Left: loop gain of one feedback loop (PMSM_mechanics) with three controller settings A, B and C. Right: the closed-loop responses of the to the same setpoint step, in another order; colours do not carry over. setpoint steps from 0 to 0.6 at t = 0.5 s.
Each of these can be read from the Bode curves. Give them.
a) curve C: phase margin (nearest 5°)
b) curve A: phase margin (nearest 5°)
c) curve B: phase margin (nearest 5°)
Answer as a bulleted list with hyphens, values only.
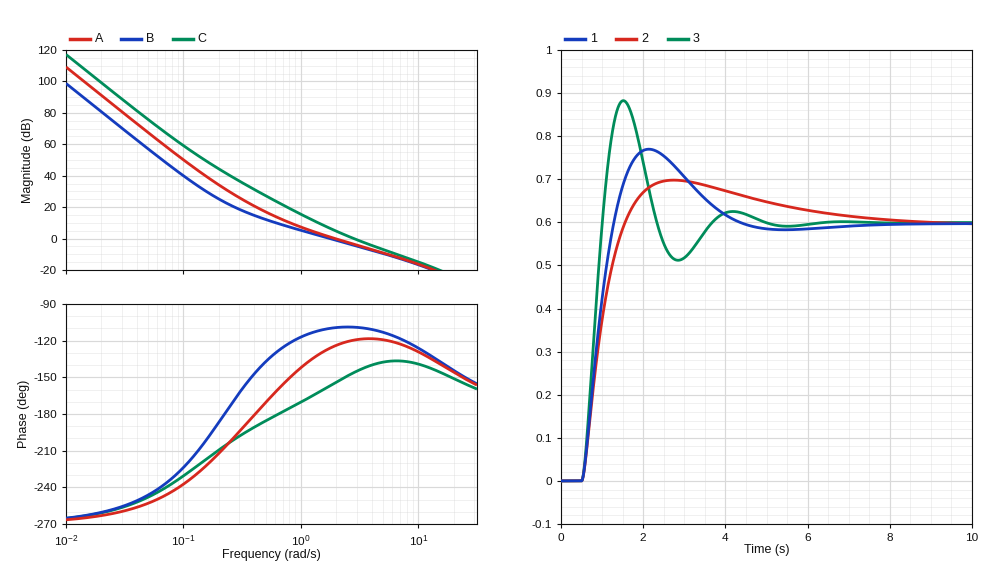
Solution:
- 35°
- 55°
- 70°
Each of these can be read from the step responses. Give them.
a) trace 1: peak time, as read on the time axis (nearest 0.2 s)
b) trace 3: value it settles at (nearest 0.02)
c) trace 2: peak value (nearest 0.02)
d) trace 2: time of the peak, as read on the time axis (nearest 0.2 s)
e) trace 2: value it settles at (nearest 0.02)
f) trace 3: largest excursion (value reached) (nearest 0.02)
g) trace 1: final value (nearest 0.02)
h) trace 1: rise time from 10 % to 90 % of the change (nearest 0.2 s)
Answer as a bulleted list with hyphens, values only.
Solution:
- 2.2 s
- 0.60
- 0.70
- 2.8 s
- 0.60
- 0.88
- 0.60
- 0.6 s
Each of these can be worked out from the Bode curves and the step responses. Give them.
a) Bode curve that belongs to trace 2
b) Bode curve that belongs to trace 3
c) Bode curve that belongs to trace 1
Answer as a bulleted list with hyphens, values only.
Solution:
- B
- C
- A
